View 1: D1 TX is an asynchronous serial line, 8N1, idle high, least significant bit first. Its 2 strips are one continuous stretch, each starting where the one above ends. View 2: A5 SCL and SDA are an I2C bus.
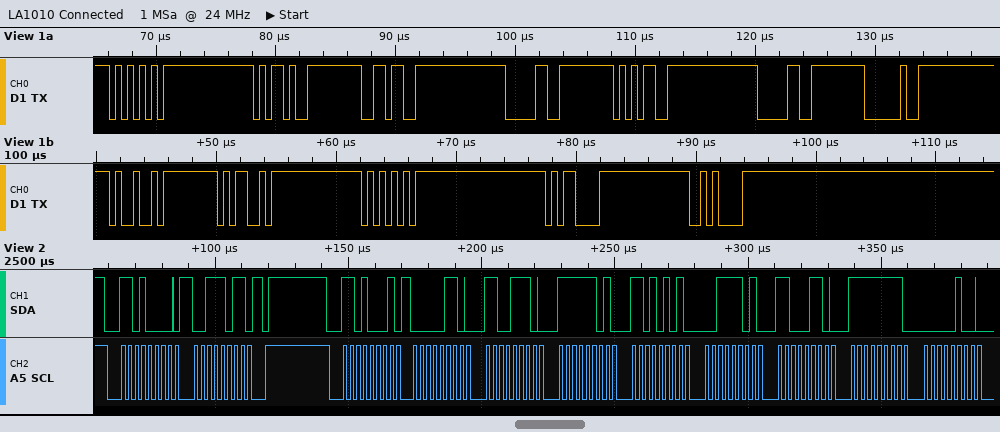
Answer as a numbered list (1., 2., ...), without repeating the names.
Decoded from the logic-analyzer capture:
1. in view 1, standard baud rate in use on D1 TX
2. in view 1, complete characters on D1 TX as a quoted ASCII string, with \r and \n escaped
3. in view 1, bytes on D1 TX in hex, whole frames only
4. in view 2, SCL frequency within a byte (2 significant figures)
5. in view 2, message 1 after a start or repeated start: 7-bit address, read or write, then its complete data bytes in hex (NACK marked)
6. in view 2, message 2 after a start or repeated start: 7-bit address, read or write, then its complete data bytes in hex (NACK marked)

1. 2000000 baud
2. "U-6050 IMU\r\n"
3. 55 2D 36 30 35 30 20 49 4D 55 0D 0A
4. 400 kHz
5. 0x68 write: 3B
6. 0x68 read: 06 CE FD D5 3D C6 FF 04
